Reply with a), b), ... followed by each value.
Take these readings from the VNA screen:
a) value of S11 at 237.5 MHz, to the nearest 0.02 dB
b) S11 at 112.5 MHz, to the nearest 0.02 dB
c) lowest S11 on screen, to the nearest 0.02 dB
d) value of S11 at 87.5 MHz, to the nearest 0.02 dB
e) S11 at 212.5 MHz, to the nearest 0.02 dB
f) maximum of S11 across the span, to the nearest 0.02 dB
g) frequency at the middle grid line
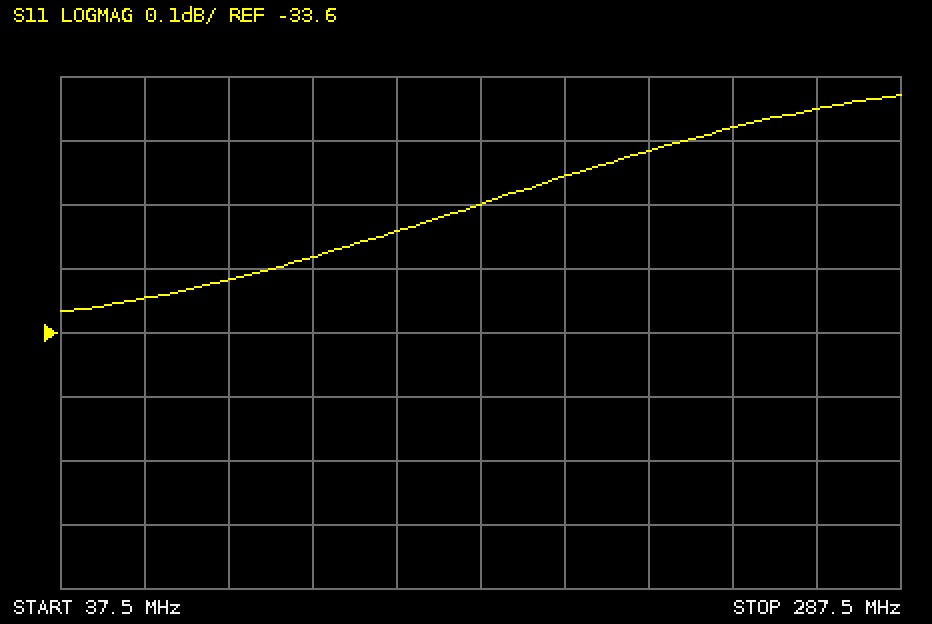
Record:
a) -33.28 dB
b) -33.48 dB
c) -33.56 dB
d) -33.52 dB
e) -33.32 dB
f) -33.22 dB
g) 162.5 MHz
